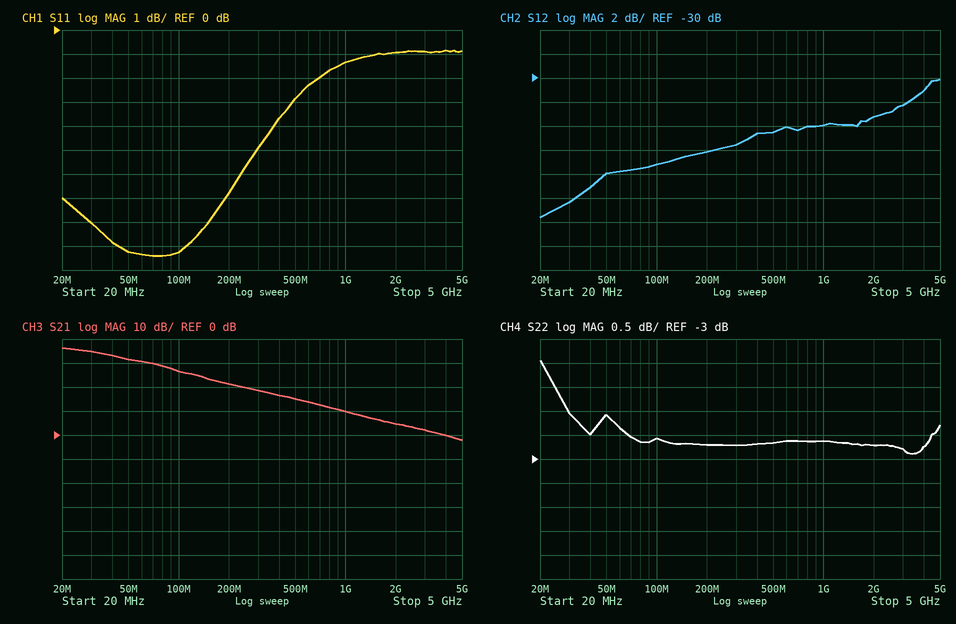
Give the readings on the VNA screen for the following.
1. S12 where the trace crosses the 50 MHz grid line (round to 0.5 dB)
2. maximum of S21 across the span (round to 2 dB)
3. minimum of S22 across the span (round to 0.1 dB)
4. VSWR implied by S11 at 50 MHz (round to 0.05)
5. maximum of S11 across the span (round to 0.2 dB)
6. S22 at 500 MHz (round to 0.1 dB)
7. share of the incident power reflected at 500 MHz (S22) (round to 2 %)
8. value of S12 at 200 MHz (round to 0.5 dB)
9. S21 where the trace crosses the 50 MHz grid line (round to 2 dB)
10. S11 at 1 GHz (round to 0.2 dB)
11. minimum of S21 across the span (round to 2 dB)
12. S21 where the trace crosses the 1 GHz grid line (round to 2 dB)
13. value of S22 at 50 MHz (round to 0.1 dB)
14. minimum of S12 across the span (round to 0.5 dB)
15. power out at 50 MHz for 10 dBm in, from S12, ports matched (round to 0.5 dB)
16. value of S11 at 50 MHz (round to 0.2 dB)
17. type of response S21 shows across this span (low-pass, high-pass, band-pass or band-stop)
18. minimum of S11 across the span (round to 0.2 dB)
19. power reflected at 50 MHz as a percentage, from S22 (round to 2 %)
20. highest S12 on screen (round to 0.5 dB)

-38.0 dB
36 dB
-2.9 dB
2.05
-0.8 dB
-2.7 dB
54 %
-36.0 dB
32 dB
-1.4 dB
-2 dB
10 dB
-2.1 dB
-41.5 dB
-28.0 dBm
-9.2 dB
low-pass
-9.4 dB
62 %
-30.0 dB
